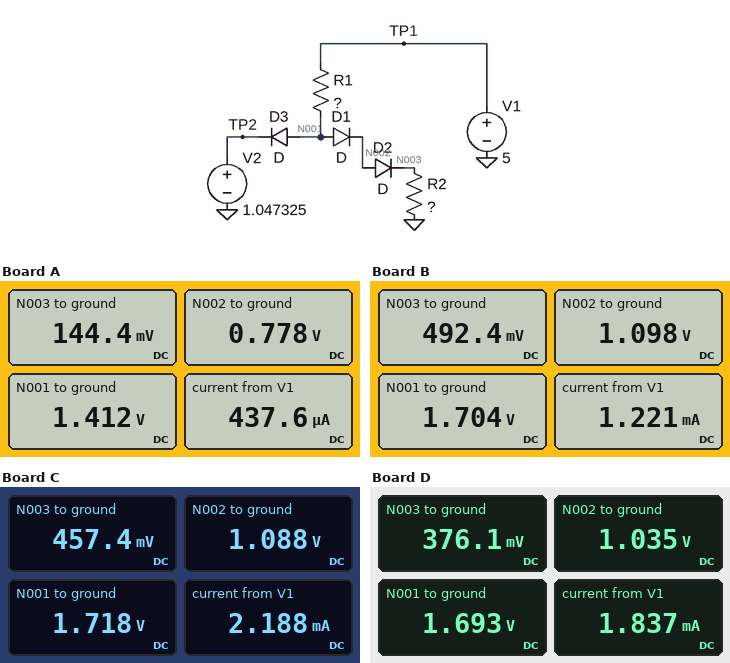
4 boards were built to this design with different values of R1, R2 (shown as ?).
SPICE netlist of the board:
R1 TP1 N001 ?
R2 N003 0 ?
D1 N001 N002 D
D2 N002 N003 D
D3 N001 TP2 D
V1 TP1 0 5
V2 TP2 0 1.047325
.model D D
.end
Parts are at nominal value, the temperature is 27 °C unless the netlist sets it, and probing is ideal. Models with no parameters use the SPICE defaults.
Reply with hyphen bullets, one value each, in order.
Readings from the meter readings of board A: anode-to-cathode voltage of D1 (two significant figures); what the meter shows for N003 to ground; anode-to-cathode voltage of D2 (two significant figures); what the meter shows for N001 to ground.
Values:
- 630 mV
- 144.4 mV
- 630 mV
- 1.412 V
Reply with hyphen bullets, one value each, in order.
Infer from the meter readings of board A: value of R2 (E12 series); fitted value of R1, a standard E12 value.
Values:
- 330 Ω
- 8.2 kΩ
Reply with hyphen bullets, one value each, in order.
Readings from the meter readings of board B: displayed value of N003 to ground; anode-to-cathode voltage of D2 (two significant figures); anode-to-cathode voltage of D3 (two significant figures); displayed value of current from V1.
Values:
- 492.4 mV
- 610 mV
- 660 mV
- 1.221 mA
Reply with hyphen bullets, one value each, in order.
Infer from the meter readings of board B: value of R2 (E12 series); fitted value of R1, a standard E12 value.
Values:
- 3.3 kΩ
- 2.7 kΩ
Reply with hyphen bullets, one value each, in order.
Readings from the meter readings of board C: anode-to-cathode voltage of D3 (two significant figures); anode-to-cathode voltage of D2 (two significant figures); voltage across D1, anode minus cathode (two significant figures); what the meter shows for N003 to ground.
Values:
- 670 mV
- 630 mV
- 630 mV
- 457.4 mV
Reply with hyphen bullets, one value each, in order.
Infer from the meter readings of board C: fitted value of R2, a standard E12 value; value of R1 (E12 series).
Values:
- 1.2 kΩ
- 1.5 kΩ
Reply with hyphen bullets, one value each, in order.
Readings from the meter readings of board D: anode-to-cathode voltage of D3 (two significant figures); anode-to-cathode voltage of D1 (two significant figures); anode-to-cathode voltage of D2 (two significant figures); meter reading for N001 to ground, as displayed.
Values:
- 650 mV
- 660 mV
- 660 mV
- 1.693 V
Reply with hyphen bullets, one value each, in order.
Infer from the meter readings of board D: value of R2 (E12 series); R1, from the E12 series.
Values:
- 330 Ω
- 1.8 kΩ
